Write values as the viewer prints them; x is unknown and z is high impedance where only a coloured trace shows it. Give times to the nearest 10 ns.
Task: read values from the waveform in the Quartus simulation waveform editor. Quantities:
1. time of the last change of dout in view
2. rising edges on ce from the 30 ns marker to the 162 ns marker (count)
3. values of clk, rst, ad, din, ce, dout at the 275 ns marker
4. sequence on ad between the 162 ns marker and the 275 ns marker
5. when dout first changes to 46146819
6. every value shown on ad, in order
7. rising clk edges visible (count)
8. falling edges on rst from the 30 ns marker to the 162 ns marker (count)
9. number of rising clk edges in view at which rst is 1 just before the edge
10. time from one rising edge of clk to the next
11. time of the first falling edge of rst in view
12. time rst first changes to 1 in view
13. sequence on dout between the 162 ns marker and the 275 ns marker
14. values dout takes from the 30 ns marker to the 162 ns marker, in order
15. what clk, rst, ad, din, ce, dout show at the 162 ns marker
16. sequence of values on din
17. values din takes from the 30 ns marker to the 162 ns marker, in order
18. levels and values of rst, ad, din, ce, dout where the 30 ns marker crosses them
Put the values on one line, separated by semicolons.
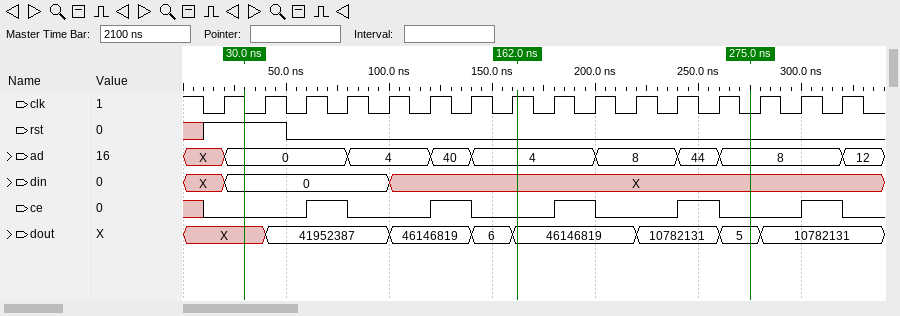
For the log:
280 ns; 2; clk=0, rst=0, ad=8, din=X, ce=0, dout=5; 4, 8, 44, 8; 100 ns; X, 0, 4, 40, 4, 8, 44, 8, 12; 16; 1; 2; 20 ns; 50 ns; 10 ns; 46146819, 10782131, 5; X, 41952387, 46146819, 6, 46146819; clk=1, rst=0, ad=4, din=X, ce=0, dout=46146819; X, 0, X; 0, X; rst=1, ad=0, din=0, ce=0, dout=X
